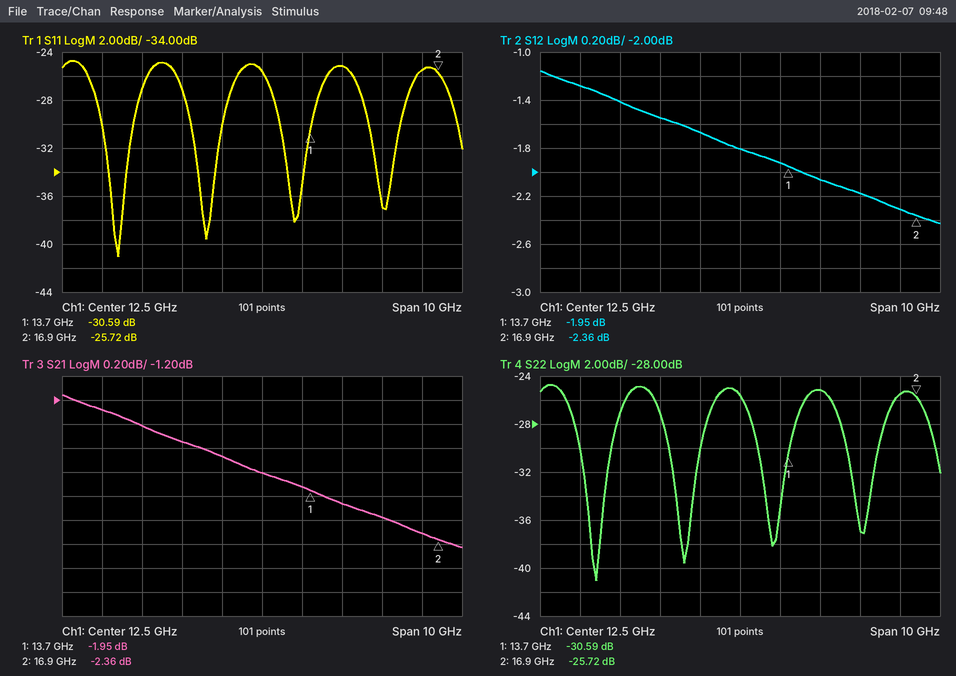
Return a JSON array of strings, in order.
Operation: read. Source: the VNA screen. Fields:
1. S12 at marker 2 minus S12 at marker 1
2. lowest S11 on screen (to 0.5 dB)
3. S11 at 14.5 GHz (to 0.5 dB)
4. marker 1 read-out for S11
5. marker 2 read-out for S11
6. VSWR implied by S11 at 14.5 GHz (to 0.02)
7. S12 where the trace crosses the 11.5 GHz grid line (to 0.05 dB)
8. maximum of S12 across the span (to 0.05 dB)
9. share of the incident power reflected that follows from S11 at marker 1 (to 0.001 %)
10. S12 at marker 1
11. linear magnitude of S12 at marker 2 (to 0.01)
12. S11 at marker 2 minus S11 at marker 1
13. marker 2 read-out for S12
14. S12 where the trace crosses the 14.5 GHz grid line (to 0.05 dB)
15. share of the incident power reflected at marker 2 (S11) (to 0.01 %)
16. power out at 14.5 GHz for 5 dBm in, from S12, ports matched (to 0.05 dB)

["-0.41 dB", "-41.0 dB", "-25.0 dB", "-30.59 dB", "-25.72 dB", "1.12", "-1.65 dB", "-1.15 dB", "0.087 %", "-1.95 dB", "0.76", "4.87 dB", "-2.36 dB", "-2.05 dB", "0.27 %", "2.95 dBm"]
